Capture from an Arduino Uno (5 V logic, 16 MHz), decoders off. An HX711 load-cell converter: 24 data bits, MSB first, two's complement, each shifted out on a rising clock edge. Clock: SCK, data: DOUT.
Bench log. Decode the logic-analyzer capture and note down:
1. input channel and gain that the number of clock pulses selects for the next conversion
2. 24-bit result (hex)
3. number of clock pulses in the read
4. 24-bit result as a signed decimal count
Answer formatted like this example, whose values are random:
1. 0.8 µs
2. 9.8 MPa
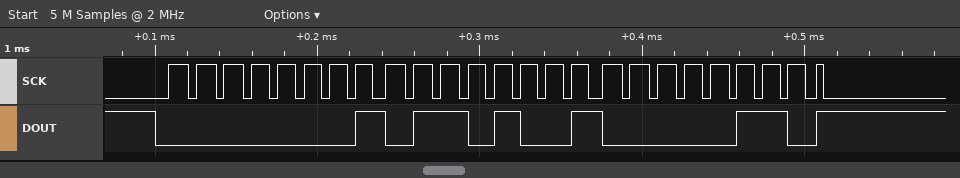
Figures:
1. channel A, gain 128
2. 0x016906
3. 25
4. 92422
